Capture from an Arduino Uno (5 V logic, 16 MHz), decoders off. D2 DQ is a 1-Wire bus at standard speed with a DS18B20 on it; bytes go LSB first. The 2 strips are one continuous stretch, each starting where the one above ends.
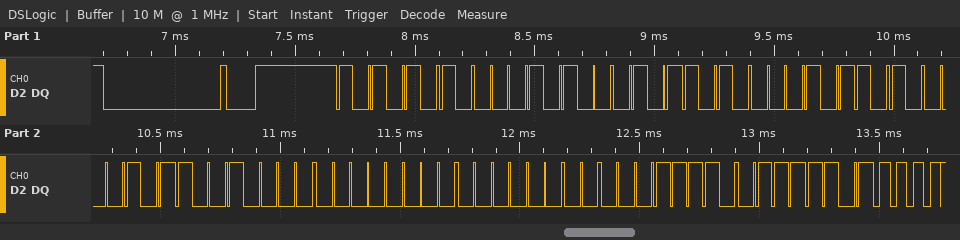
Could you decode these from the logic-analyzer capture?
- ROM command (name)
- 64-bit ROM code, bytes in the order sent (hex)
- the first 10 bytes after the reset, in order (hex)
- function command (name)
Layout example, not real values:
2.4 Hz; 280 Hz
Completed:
Match ROM; 28 5A 68 A1 09 00 00 78; 55 28 5A 68 A1 09 00 00 78 BE; Read Scratchpad
